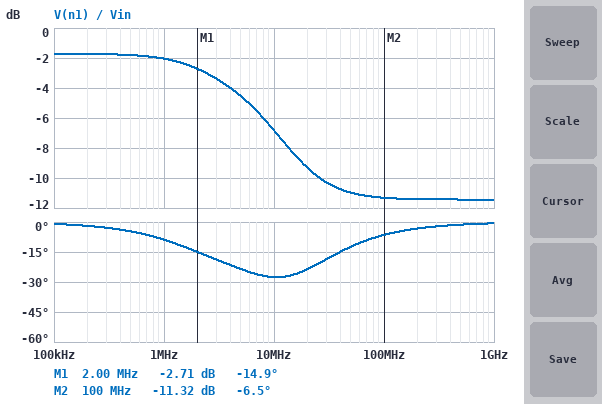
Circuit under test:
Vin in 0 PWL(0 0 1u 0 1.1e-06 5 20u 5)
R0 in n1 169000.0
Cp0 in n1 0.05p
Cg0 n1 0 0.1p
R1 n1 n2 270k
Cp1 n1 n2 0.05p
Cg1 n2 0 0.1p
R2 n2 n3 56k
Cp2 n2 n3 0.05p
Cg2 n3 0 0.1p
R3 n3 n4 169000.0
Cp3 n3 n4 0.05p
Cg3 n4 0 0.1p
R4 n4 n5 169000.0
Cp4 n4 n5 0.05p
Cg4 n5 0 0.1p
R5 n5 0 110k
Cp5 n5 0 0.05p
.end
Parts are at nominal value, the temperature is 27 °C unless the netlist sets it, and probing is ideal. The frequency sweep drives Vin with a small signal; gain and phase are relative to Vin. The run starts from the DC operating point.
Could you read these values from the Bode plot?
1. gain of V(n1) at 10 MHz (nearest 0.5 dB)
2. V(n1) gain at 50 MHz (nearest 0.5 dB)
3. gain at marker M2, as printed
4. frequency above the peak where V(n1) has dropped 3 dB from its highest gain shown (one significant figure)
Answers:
-7.0 dB
-11.0 dB
-11.32 dB
5 MHz
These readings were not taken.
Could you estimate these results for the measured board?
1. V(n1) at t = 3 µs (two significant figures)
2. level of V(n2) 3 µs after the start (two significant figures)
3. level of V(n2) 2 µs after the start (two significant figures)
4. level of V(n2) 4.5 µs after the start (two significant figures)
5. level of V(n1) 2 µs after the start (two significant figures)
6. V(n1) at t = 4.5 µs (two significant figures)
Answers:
4.1 V
2.7 V
2.7 V
2.7 V
4.1 V
4.1 V
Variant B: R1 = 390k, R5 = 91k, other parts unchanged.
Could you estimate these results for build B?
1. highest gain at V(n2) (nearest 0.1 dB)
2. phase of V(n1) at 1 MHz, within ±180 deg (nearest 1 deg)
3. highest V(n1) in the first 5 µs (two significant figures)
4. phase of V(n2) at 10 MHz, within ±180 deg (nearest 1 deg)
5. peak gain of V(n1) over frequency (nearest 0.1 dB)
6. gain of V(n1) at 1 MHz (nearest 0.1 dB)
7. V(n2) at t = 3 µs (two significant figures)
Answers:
-6.7 dB
-8 deg
4.2 V
-43 deg
-1.5 dB
-1.8 dB
2.3 V
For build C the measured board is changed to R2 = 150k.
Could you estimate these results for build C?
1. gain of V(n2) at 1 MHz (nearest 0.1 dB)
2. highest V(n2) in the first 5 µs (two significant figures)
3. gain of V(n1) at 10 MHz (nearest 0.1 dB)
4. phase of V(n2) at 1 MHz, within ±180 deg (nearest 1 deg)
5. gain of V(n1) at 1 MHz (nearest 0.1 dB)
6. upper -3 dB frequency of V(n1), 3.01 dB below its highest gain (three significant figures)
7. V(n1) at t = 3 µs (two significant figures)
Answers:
-5.5 dB
2.9 V
-6.7 dB
-20 deg
-1.9 dB
5.36 MHz
4.2 V
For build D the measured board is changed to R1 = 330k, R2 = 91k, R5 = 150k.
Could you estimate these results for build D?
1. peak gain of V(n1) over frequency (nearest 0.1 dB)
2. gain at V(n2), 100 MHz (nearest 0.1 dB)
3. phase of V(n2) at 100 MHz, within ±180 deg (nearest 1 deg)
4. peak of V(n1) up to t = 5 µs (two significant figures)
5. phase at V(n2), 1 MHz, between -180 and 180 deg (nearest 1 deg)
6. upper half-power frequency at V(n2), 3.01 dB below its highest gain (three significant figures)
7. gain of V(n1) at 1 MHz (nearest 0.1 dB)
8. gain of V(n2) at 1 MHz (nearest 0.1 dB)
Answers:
-1.5 dB
-22.8 dB
-8 deg
4.2 V
-22 deg
2.08 MHz
-1.8 dB
-6.3 dB
